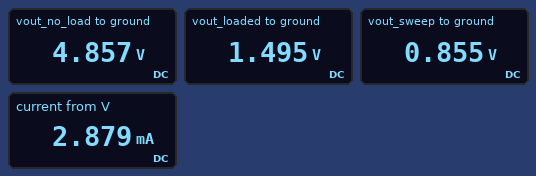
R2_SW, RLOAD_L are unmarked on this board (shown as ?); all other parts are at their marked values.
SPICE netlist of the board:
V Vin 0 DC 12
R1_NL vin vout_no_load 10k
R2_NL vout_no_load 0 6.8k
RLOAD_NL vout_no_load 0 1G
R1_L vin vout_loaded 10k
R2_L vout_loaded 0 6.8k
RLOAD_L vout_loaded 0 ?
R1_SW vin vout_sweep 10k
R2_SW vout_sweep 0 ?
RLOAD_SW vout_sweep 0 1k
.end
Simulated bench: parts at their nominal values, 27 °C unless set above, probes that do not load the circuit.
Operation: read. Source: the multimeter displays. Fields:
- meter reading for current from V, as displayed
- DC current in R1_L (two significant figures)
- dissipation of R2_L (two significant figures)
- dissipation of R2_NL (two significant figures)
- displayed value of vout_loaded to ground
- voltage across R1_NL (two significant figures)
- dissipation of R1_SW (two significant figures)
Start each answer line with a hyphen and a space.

- 2.879 mA
- 1.1 mA
- 330 µW
- 3.5 mW
- 1.495 V
- 7.1 V
- 12 mW
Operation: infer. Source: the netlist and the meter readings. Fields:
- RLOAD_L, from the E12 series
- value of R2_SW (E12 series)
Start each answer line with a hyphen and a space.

- 1.8 kΩ
- 3.3 kΩ
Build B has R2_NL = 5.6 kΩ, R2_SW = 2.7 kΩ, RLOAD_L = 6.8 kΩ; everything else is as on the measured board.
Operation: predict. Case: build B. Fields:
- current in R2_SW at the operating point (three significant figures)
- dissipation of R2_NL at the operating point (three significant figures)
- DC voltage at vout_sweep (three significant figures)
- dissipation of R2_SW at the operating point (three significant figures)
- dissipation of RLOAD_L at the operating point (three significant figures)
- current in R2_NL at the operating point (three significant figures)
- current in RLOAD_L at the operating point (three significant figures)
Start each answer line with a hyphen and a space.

- 302 µA
- 3.31 mW
- 816 mV
- 247 µW
- 1.36 mW
- 769 µA
- 448 µA
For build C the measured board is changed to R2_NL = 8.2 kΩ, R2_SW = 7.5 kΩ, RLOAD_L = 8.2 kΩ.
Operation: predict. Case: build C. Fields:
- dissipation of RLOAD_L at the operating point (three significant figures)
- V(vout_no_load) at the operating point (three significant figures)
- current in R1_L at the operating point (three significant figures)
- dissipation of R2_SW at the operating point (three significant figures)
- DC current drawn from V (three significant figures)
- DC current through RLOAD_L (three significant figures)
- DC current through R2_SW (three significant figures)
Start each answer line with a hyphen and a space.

- 1.29 mW
- 5.41 V
- 875 µA
- 126 µW
- 2.64 mA
- 397 µA
- 130 µA
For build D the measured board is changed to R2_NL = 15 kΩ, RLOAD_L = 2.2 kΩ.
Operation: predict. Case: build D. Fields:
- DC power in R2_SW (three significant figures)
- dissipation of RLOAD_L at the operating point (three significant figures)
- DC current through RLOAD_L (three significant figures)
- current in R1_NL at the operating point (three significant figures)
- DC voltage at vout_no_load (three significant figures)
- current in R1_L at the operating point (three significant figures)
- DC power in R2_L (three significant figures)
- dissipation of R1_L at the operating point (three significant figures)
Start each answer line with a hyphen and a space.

- 222 µW
- 1.33 mW
- 777 µA
- 480 µA
- 7.20 V
- 1.03 mA
- 430 µW
- 10.6 mW
